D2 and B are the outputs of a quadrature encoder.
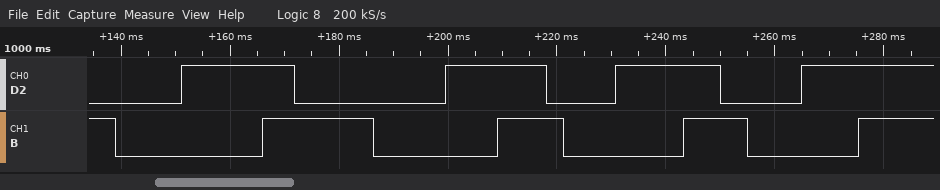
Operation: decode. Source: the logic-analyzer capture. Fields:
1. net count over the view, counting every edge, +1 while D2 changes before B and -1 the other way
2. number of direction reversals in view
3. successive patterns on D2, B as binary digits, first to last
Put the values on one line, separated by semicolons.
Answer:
+15; 0; 01 00 10 11 01 00 10 11 01 00 10 11 01 00 10 11
